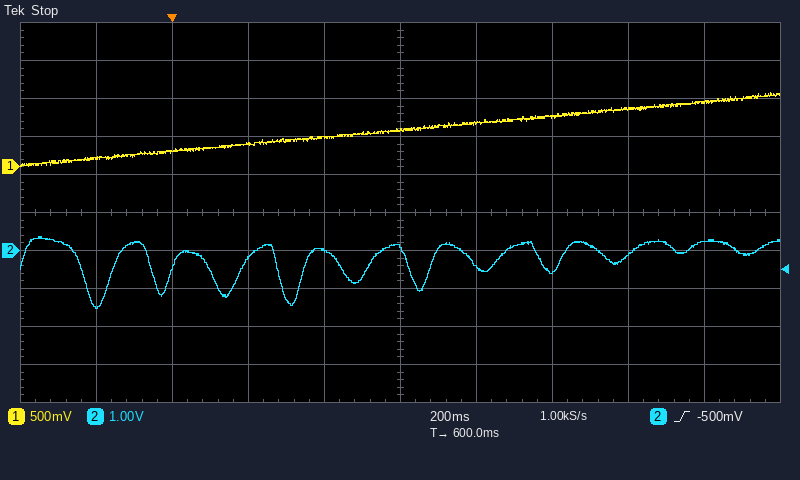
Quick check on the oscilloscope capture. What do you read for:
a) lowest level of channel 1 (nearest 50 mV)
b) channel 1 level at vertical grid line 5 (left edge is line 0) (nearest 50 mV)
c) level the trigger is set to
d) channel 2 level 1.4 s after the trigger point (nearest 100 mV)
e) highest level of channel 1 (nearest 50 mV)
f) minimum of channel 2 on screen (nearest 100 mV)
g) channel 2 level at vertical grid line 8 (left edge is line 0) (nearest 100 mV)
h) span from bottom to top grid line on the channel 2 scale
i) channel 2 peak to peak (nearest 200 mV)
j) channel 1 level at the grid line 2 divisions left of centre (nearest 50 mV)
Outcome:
0 mV
500 mV
-500 mV
200 mV
1.00 V
-1.5 V
-100 mV
10 V
1.8 V
300 mV
